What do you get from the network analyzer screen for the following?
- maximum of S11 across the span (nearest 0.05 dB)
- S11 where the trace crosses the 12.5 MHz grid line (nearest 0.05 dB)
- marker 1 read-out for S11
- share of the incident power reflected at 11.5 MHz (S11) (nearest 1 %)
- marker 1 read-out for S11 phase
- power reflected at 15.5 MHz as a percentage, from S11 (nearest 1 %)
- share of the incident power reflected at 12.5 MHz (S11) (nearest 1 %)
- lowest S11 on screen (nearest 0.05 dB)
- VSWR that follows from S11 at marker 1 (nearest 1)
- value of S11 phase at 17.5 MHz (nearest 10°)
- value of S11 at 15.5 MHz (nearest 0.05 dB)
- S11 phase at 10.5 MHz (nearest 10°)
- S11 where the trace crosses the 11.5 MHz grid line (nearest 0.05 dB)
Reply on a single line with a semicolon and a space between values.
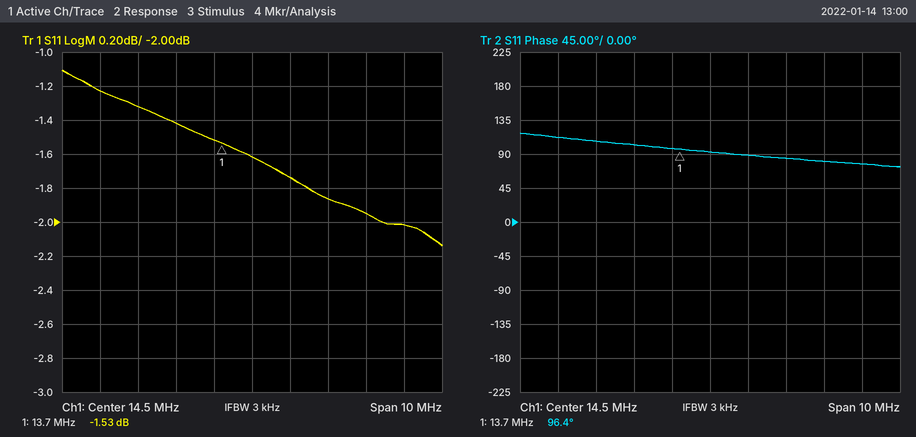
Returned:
-1.10 dB; -1.40 dB; -1.53 dB; 74 %; 96.4°; 67 %; 72 %; -2.15 dB; 11; 80°; -1.75 dB; 110°; -1.30 dB
